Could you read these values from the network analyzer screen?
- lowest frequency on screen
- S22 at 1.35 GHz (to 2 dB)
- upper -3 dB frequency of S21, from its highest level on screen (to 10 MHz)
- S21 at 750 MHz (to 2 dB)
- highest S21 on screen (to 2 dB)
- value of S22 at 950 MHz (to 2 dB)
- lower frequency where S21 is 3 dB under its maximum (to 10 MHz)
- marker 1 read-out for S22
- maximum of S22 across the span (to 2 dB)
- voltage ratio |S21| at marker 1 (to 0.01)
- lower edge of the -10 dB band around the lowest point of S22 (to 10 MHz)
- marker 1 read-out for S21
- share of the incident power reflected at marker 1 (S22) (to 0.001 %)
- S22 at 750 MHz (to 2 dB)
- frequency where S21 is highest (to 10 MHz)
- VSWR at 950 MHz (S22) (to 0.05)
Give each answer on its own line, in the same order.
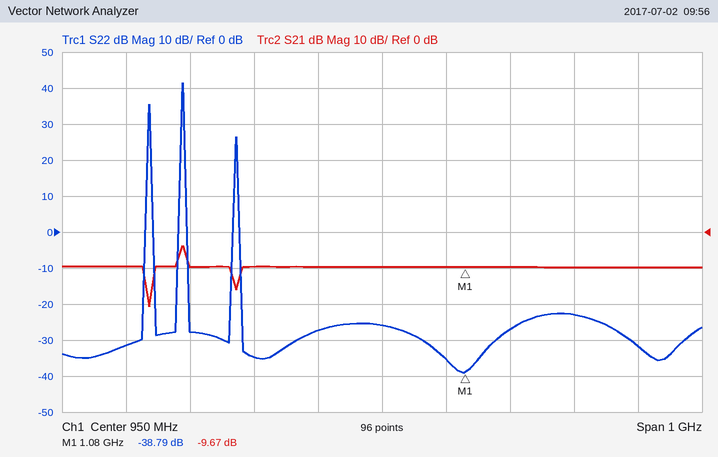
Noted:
450 MHz
-32 dB
640 MHz
-10 dB
-4 dB
-26 dB
630 MHz
-38.79 dB
42 dB
0.33
730 MHz
-9.67 dB
0.013 %
-34 dB
640 MHz
1.10
